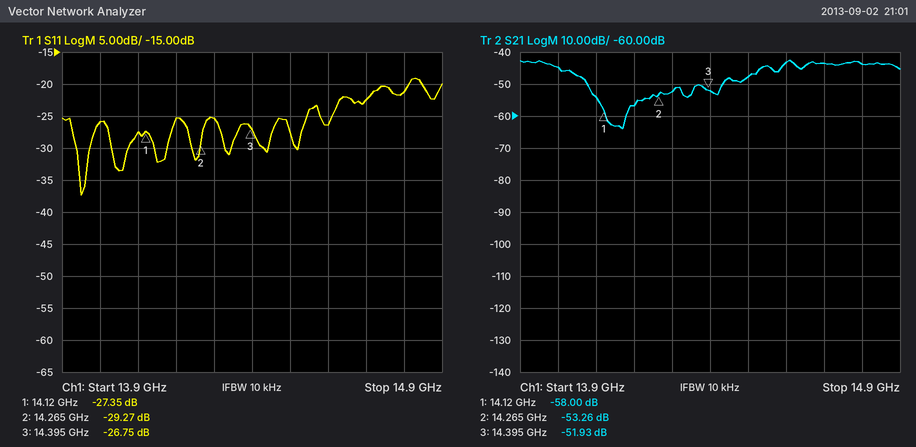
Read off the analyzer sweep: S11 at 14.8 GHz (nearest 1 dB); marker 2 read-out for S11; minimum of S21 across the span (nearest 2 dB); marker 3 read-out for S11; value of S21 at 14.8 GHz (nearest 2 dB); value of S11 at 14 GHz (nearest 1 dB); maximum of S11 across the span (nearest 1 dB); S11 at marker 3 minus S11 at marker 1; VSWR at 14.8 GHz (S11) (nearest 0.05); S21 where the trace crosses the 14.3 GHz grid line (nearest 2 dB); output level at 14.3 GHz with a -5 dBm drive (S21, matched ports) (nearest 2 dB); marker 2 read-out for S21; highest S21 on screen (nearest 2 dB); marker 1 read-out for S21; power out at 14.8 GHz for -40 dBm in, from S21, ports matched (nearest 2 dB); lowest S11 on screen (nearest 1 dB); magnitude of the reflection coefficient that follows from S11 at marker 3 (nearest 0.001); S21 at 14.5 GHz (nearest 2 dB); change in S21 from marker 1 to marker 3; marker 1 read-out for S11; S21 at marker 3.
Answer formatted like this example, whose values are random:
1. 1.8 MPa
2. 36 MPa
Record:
1. -21 dB
2. -29.27 dB
3. -64 dB
4. -26.75 dB
5. -44 dB
6. -26 dB
7. -19 dB
8. 0.60 dB
9. 1.20
10. -52 dB
11. -58 dBm
12. -53.26 dB
13. -42 dB
14. -58.00 dB
15. -84 dBm
16. -37 dB
17. 0.046
18. -48 dB
19. 6.07 dB
20. -27.35 dB
21. -51.93 dB
